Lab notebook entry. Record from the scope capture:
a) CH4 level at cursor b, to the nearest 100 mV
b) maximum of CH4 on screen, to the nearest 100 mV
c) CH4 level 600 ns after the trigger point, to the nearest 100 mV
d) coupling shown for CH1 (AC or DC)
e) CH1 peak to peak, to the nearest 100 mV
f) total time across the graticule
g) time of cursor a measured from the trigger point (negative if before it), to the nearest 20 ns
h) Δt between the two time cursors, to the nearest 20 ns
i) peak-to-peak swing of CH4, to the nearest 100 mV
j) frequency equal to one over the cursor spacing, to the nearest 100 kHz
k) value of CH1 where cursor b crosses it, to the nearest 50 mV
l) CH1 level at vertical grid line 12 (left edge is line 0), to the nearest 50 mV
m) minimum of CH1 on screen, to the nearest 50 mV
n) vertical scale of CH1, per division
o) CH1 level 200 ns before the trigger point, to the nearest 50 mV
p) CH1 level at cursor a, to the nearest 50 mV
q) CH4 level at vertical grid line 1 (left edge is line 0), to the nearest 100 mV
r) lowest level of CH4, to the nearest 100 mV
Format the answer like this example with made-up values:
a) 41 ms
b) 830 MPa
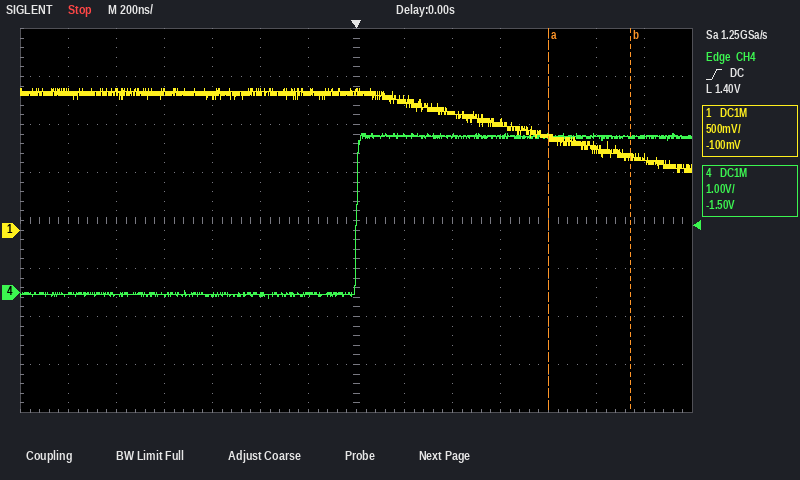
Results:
a) 3.2 V
b) 3.3 V
c) 3.2 V
d) DC
e) 900 mV
f) 2.8 µs
g) +800 ns
h) 340 ns
i) 3.4 V
j) 2.9 MHz
k) 750 mV
l) 850 mV
m) 600 mV
n) 500 mV
o) 1.40 V
p) 950 mV
q) 0.0 V
r) -100 mV
